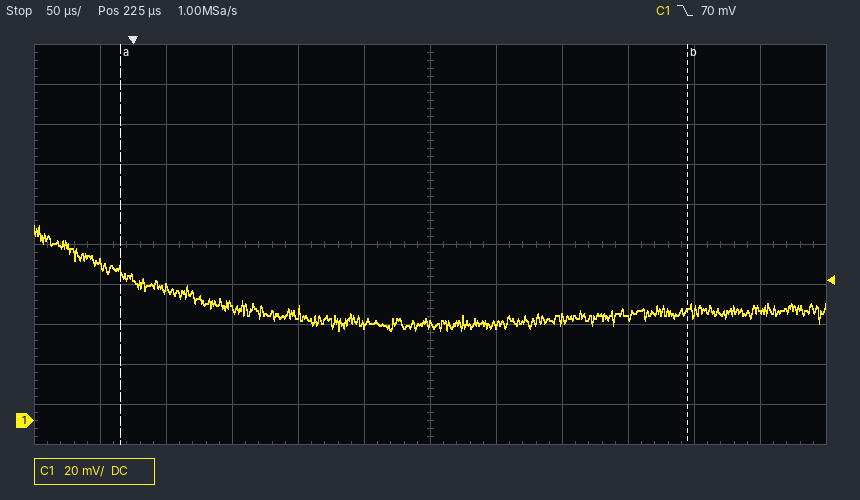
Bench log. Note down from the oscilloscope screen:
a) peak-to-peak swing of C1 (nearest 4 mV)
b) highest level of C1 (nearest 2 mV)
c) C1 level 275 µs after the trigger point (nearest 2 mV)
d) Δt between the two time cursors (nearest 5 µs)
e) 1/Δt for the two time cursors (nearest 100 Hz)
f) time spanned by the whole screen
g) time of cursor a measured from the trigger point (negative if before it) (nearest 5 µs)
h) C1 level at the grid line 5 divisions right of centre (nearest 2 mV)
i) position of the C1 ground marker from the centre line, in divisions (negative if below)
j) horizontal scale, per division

52 mV
98 mV
48 mV
430 µs
2.3 kHz
600 µs
-10 µs
56 mV
-4.4 div
50 µs
